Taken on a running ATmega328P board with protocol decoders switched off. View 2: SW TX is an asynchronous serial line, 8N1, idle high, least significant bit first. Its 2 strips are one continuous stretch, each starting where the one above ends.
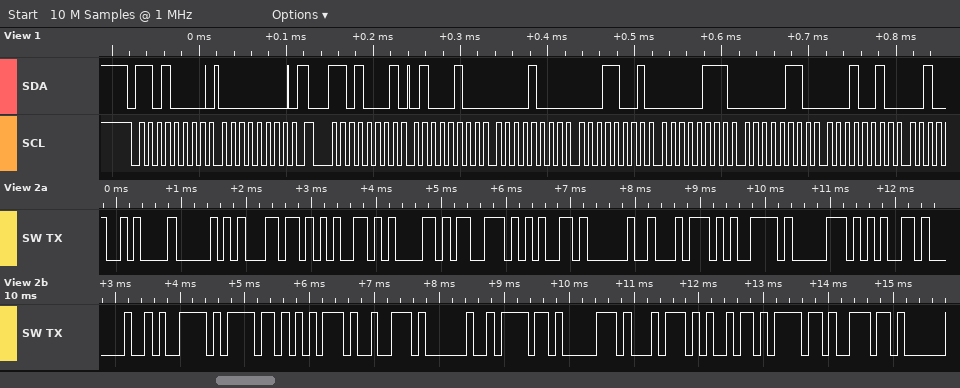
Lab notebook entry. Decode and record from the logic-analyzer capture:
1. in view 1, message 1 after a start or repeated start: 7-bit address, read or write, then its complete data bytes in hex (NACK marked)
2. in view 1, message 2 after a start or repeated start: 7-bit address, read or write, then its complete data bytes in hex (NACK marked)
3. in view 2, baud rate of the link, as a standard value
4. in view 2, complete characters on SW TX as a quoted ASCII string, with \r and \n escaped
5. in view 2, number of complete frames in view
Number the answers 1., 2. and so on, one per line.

1. 0x68 write: 00
2. 0x68 read: 44 08 19 07 06 12
3. 9600 baud
4. "\nPlease type your option"
5. 24
